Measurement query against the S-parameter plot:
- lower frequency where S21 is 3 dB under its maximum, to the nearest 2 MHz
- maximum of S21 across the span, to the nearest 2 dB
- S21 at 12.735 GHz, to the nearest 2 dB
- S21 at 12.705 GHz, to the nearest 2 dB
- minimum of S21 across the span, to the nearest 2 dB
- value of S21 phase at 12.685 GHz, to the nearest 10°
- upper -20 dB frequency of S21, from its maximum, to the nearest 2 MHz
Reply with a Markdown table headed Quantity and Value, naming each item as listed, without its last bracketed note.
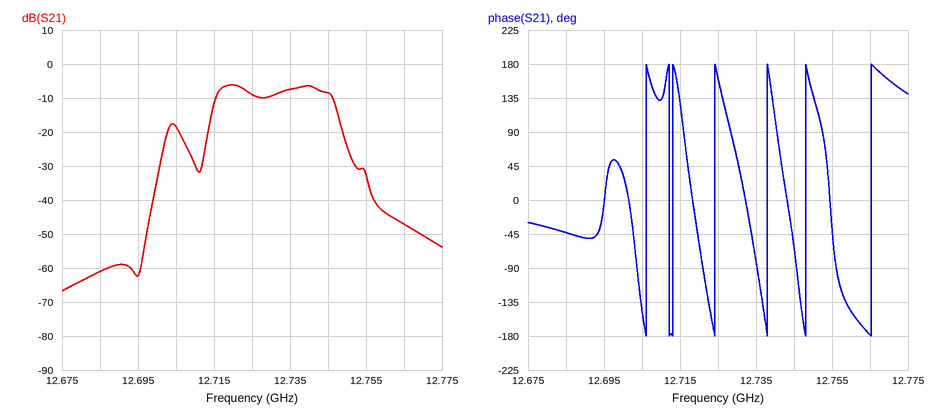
| Quantity | Value |
|---|---|
| lower frequency where S21 is 3 dB under its maximum, to the nearest 2 MHz | 12.716 GHz |
| maximum of S21 across the span, to the nearest 2 dB | -6 dB |
| S21 at 12.735 GHz, to the nearest 2 dB | -8 dB |
| S21 at 12.705 GHz, to the nearest 2 dB | -18 dB |
| minimum of S21 across the span, to the nearest 2 dB | -66 dB |
| value of S21 phase at 12.685 GHz, to the nearest 10° | -40° |
| upper -20 dB frequency of S21, from its maximum, to the nearest 2 MHz | 12.750 GHz |
